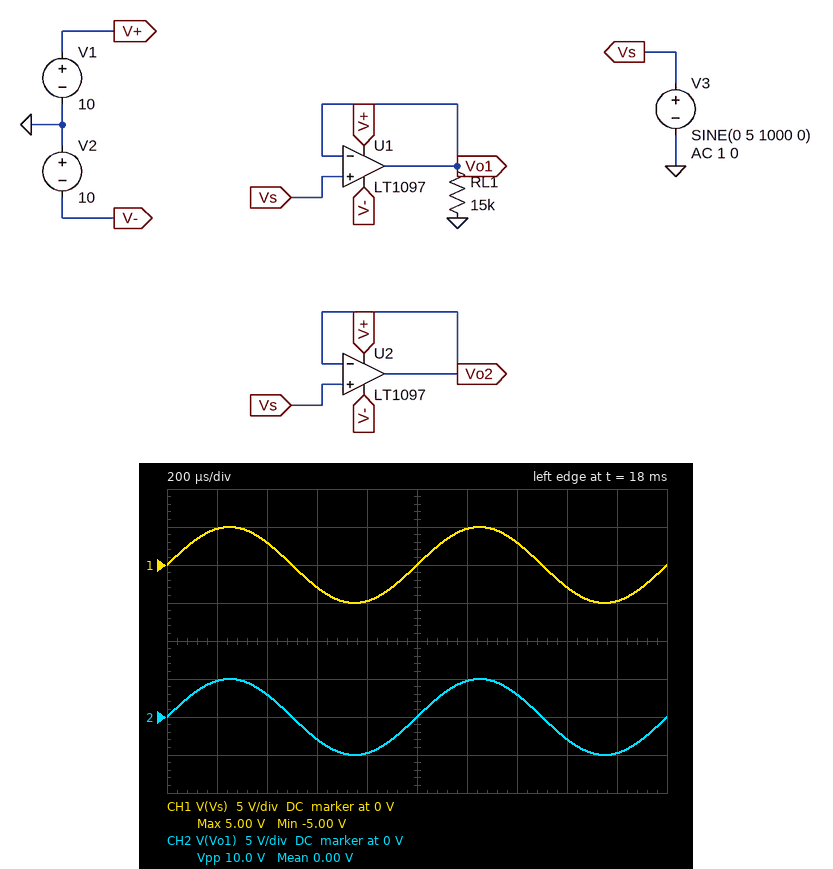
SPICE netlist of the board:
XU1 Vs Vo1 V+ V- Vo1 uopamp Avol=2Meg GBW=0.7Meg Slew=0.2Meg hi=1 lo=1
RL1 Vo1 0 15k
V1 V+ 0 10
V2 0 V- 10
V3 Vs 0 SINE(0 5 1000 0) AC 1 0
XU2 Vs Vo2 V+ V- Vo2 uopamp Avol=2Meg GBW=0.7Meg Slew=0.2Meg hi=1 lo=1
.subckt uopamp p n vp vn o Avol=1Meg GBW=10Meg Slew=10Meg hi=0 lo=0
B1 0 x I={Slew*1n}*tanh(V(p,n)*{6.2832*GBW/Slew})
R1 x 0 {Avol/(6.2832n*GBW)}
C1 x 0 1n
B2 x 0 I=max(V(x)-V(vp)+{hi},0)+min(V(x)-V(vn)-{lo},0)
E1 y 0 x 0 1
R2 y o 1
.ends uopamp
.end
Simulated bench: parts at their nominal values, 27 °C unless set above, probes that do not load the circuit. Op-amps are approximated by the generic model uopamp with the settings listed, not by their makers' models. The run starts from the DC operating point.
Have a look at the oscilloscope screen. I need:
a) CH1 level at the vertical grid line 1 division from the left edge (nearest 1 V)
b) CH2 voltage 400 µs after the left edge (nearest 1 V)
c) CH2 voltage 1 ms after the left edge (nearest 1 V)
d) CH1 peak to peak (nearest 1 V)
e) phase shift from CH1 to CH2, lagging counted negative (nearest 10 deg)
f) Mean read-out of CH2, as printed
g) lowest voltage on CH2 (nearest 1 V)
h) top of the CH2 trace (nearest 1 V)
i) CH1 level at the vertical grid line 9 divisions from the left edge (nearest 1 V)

5 V
3 V
0 V
10 V
0 deg
0.00 V
-5 V
5 V
-5 V
